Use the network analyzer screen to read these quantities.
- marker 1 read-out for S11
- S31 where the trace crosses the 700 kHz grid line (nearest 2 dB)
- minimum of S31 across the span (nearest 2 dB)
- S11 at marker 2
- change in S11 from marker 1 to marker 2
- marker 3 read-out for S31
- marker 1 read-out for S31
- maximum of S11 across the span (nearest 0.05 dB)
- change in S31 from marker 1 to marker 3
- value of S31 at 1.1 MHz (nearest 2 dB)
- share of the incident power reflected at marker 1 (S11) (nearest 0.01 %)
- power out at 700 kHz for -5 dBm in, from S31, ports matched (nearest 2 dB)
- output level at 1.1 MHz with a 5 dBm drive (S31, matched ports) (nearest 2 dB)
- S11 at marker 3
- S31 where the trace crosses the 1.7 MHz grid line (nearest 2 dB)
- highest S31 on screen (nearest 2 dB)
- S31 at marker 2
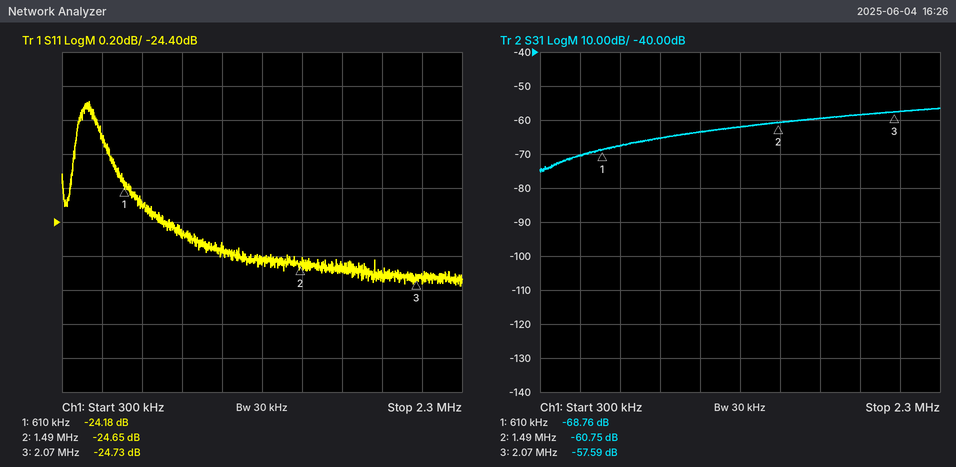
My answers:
-24.18 dB
-68 dB
-76 dB
-24.65 dB
-0.47 dB
-57.59 dB
-68.76 dB
-23.70 dB
11.17 dB
-64 dB
0.38 %
-72 dBm
-58 dBm
-24.73 dB
-60 dB
-56 dB
-60.75 dB
